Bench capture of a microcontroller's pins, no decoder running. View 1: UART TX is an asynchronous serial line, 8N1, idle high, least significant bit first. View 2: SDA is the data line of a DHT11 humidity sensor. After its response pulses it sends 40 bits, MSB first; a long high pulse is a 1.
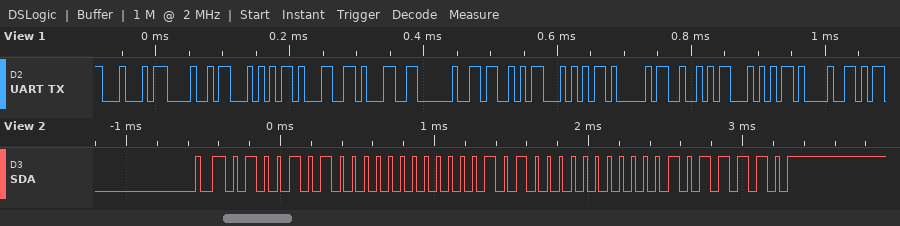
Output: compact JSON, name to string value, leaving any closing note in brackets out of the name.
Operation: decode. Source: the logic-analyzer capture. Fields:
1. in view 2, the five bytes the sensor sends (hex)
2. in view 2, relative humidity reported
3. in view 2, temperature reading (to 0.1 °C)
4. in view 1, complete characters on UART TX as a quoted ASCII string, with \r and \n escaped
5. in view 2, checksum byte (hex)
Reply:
{"in view 2, the five bytes the sensor sends": "4A 00 14 00 5E", "in view 2, relative humidity reported": "74 %", "in view 2, temperature reading": "20.0 °C", "in view 1, complete characters on UART TX as a quoted ASCII string, with \\r and \\n escaped": "\"DHT11 START!\"", "in view 2, checksum byte": "0x5E"}
